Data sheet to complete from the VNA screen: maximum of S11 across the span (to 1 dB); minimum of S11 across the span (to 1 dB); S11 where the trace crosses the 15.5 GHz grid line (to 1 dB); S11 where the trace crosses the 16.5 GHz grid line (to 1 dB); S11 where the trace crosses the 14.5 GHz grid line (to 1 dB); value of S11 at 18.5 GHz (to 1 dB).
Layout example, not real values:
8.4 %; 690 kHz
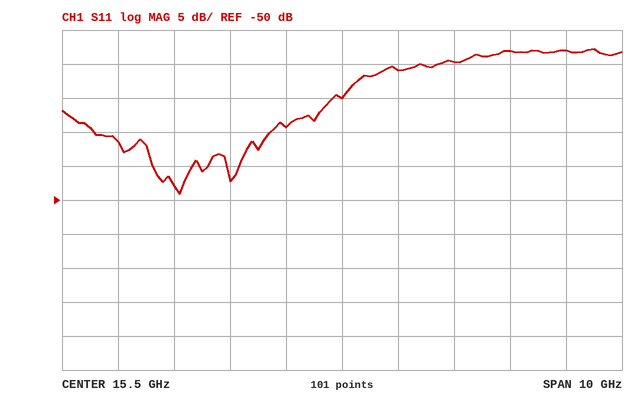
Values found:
-28 dB; -49 dB; -35 dB; -31 dB; -39 dB; -28 dB
